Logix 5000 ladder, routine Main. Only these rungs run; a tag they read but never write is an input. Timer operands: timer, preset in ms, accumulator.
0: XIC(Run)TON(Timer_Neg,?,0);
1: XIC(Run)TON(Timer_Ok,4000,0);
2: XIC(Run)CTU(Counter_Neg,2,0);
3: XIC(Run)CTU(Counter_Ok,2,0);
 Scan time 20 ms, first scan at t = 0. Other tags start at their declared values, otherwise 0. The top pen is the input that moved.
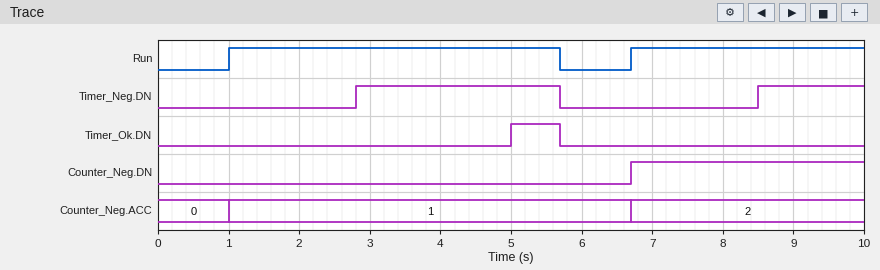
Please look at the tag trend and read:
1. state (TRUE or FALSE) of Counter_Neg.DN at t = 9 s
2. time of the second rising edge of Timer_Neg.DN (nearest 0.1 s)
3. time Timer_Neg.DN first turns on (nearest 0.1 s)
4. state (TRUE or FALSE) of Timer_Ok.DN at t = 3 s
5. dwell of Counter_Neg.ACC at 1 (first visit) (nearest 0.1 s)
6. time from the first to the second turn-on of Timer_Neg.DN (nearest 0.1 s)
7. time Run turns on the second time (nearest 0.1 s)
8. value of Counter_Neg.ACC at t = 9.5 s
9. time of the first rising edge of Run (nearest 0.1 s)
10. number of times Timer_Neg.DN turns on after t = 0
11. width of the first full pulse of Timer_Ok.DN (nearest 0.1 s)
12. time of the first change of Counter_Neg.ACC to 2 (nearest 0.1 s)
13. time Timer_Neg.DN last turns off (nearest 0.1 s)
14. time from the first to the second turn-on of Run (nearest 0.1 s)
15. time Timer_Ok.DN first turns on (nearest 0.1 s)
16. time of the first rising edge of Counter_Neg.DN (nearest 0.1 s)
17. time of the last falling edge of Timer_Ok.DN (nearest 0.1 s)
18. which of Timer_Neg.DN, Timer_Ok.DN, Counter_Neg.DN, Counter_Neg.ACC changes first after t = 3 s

TRUE
8.5 s
2.8 s
FALSE
5.7 s
5.7 s
6.7 s
2
1.0 s
2
0.7 s
6.7 s
5.7 s
5.7 s
5.0 s
6.7 s
5.7 s
Timer_Ok.DN
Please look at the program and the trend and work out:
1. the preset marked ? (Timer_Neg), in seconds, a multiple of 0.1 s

1.8 s
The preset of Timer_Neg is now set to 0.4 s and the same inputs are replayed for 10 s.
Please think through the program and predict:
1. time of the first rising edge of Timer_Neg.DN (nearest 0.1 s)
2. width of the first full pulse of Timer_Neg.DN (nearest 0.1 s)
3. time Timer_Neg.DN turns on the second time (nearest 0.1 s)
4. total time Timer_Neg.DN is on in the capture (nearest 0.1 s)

1.4 s
4.3 s
7.1 s
7.2 s
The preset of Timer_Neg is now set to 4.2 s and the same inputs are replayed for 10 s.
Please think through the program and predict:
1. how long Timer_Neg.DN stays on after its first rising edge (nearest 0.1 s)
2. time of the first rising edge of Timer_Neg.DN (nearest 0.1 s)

0.5 s
5.2 s
